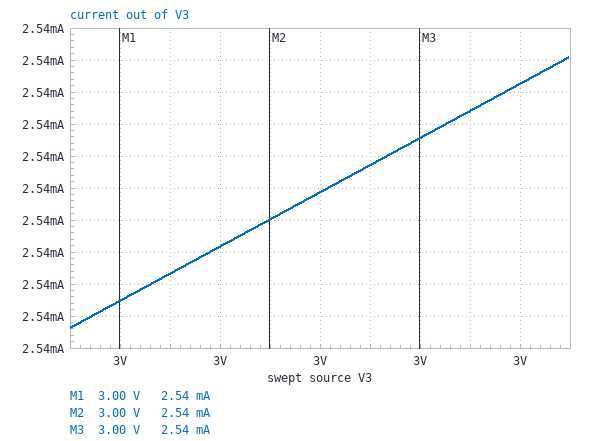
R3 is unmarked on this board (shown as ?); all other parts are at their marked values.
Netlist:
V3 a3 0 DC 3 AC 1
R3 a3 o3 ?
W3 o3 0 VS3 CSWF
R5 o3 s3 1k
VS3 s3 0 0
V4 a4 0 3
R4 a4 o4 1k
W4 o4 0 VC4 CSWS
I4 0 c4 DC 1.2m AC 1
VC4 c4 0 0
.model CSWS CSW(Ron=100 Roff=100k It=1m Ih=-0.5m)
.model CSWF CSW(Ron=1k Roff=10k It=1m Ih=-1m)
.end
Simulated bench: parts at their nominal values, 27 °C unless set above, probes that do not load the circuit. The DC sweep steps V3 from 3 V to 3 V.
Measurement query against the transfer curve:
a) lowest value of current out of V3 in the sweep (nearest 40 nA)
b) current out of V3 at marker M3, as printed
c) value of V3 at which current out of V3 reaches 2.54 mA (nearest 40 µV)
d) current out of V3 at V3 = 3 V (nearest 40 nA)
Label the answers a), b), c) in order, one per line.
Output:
a) 2.54152 mA
b) 2.54 mA
c) 2.99956 V
d) 2.54204 mA
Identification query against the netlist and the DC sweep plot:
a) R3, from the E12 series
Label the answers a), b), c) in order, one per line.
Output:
a) 680 Ω
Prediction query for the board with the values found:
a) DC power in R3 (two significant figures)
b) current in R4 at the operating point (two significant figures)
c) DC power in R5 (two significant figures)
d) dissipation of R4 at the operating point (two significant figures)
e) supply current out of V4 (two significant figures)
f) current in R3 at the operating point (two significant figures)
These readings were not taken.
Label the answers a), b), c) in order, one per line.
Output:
a) 4.4 mW
b) 2.7 mA
c) 1.6 mW
d) 7.4 mW
e) 2.7 mA
f) 2.5 mA
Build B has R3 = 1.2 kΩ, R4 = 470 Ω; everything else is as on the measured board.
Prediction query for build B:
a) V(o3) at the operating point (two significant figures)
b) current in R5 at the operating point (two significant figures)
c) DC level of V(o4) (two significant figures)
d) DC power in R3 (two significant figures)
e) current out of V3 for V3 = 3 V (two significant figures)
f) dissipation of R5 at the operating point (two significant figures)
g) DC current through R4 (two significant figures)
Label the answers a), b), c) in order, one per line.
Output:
a) 880 mV
b) 880 µA
c) 530 mV
d) 3.7 mW
e) 1.8 mA
f) 780 µW
g) 5.3 mA
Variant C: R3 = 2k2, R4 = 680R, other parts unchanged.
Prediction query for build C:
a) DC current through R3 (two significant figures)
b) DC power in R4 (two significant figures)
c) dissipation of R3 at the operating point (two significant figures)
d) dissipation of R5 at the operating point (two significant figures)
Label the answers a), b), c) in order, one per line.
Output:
a) 1.1 mA
b) 10 mW
c) 2.7 mW
d) 310 µW
